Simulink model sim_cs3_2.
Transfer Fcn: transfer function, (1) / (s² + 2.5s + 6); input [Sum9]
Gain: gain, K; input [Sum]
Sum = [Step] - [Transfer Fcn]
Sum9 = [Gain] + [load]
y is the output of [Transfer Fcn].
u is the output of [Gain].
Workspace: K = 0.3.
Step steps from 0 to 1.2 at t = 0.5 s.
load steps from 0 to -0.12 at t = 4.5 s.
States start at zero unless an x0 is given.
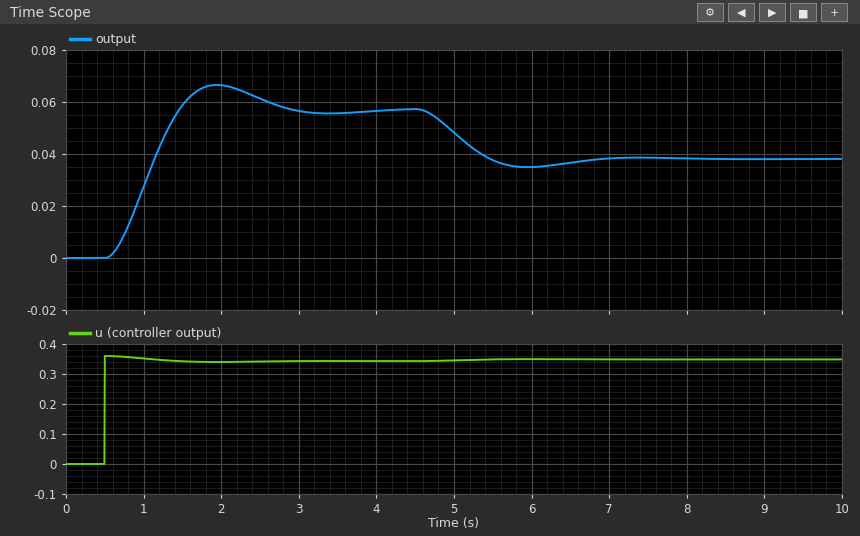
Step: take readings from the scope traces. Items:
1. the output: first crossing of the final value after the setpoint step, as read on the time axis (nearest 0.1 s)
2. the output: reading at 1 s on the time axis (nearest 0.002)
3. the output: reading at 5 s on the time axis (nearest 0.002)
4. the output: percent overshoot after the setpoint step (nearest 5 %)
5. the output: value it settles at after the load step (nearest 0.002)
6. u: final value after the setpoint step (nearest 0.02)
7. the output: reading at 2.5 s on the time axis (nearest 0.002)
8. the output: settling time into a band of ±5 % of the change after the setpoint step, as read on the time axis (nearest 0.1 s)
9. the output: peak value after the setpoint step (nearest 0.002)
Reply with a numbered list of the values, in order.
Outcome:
1. 1.5 s
2. 0.028
3. 0.048
4. 15 %
5. 0.038
6. 0.34
7. 0.062
8. 2.6 s
9. 0.066
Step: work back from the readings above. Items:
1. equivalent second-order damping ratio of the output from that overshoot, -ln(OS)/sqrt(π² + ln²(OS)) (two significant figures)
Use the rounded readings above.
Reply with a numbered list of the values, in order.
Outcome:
1. 0.52
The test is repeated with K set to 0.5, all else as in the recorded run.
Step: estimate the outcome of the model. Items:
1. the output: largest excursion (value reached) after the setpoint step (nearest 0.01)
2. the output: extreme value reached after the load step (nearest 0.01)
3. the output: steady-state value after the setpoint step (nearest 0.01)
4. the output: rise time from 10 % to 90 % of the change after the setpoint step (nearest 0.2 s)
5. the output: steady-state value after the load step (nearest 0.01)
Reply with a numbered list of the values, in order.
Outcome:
1. 0.11
2. 0.07
3. 0.09
4. 0.6 s
5. 0.07
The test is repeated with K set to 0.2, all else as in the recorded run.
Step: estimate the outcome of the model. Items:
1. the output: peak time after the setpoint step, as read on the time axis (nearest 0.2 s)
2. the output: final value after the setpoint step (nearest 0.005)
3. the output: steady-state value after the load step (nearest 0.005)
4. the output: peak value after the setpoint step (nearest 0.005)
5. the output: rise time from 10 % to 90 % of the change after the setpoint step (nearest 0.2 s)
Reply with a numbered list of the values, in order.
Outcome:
1. 2.0 s
2. 0.040
3. 0.020
4. 0.045
5. 0.6 s
